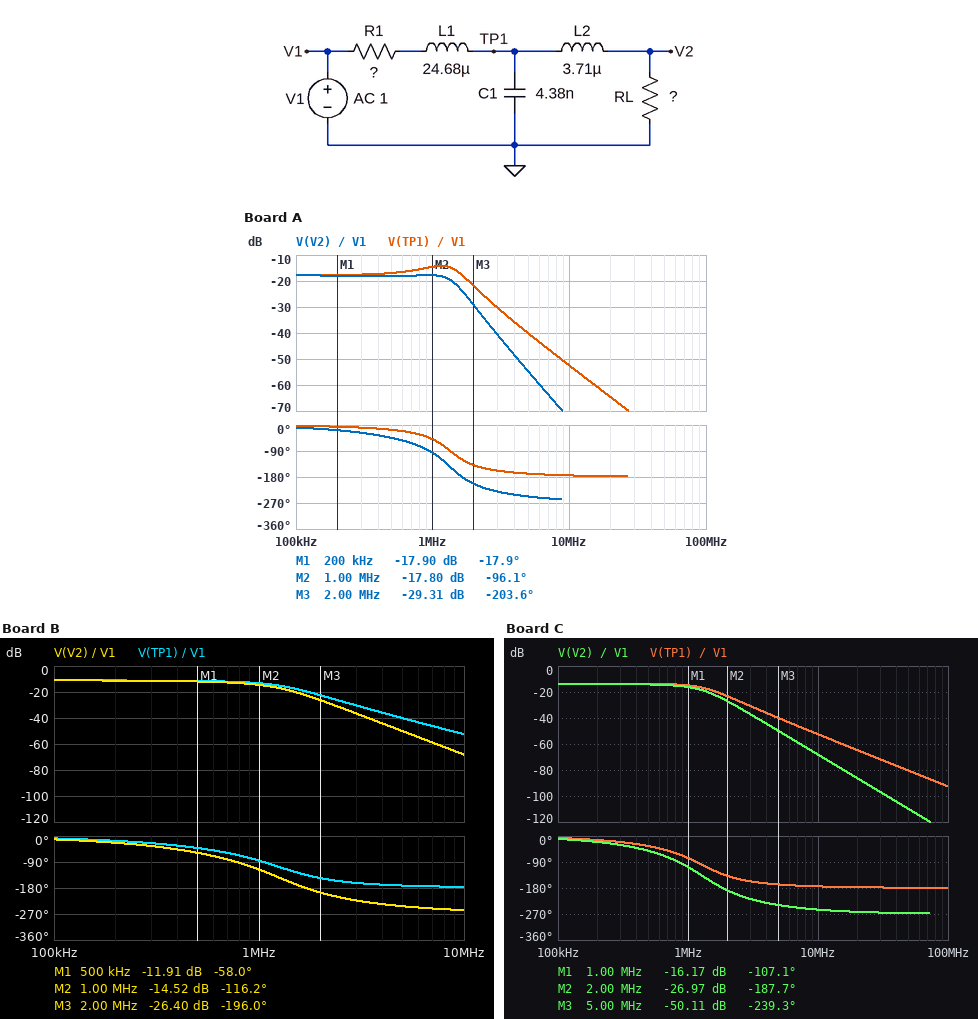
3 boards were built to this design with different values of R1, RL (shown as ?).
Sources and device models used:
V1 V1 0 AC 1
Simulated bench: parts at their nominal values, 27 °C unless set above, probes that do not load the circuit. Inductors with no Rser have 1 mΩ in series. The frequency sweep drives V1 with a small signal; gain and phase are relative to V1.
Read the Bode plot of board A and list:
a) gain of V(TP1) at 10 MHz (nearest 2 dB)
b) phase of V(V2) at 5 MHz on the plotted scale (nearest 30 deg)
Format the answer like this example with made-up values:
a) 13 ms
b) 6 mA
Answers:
a) -52 dB
b) -240 deg
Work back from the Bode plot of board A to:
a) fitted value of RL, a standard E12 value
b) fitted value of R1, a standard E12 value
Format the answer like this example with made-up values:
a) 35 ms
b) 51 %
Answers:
a) 22 Ω
b) 150 Ω
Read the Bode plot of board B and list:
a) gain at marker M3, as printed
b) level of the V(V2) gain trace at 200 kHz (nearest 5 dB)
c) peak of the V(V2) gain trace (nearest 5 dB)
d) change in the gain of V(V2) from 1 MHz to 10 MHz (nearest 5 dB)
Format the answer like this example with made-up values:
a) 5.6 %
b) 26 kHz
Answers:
a) -26.40 dB
b) -10 dB
c) -10 dB
d) -55 dB
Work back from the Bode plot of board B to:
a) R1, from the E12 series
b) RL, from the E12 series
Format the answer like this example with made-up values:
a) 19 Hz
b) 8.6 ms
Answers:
a) 100 Ω
b) 39 Ω
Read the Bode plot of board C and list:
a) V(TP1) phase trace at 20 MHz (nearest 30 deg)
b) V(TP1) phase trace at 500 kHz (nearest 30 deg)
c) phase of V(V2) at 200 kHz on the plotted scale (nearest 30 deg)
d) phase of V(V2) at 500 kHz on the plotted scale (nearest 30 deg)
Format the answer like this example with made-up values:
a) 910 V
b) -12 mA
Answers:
a) -180 deg
b) -30 deg
c) -30 deg
d) -60 deg
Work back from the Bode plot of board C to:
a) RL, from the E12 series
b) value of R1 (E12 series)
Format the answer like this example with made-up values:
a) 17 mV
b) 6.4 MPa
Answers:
a) 39 Ω
b) 150 Ω
